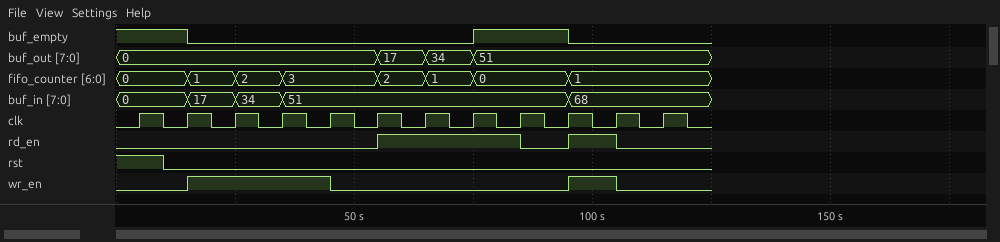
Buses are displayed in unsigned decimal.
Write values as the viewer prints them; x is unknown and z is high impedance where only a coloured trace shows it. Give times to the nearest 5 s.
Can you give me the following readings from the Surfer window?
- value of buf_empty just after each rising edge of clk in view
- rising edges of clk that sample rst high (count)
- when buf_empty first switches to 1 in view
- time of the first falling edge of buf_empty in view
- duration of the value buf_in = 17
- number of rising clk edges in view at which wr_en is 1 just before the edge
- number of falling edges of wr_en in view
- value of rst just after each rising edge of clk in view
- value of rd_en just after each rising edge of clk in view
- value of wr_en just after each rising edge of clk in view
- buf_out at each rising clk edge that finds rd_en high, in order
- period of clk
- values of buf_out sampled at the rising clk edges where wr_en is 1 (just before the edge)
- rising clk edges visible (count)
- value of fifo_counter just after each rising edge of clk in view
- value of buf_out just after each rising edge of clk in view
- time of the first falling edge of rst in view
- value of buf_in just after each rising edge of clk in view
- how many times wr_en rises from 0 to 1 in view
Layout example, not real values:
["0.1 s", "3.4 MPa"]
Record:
["1 0 0 0 0 0 0 1 1 0 0 0", "1", "75 s", "15 s", "10 s", "4", "2", "1 0 0 0 0 0 0 0 0 0 0 0", "0 0 0 0 0 1 1 1 0 1 0 0", "0 1 1 1 0 0 0 0 0 1 0 0", "17, 34, 51, 51", "10 s", "0, 0, 0, 51", "12", "0, 1, 2, 3, 3, 2, 1, 0, 0, 1, 1, 1", "0, 0, 0, 0, 0, 17, 34, 51, 51, 51, 51, 51", "10 s", "0, 17, 34, 51, 51, 51, 51, 51, 51, 68, 68, 68", "2"]
